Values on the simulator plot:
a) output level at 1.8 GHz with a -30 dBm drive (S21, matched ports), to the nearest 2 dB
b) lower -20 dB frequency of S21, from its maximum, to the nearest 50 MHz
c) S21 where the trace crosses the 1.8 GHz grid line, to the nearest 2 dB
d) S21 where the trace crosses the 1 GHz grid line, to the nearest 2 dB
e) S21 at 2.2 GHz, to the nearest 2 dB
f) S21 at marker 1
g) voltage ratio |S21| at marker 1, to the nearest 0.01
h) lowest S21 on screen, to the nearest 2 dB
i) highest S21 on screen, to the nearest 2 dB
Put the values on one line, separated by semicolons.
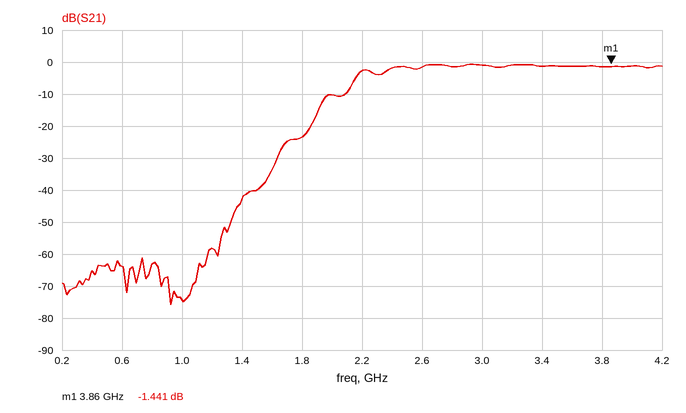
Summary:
-54 dBm; 1.85 GHz; -24 dB; -74 dB; -2 dB; -1.441 dB; 0.85; -76 dB; 0 dB
